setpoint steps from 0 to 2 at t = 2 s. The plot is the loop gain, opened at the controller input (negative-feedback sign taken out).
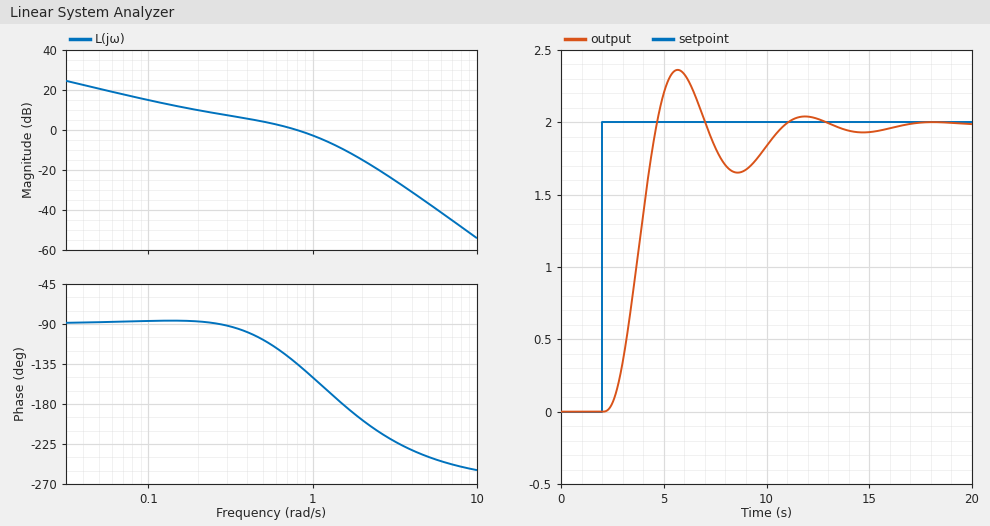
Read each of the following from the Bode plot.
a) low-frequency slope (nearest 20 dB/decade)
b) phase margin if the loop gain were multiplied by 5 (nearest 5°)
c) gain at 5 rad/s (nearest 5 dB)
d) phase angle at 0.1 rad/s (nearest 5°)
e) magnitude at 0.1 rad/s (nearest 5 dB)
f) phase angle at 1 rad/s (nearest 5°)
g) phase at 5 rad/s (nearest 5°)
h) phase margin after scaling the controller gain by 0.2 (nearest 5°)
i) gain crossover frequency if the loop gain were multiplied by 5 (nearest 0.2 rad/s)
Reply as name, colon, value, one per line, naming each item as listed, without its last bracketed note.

low-frequency slope: -20 dB/decade
phase margin if the loop gain were multiplied by 5: -15°
gain at 5 rad/s: -35 dB
phase angle at 0.1 rad/s: -85°
magnitude at 0.1 rad/s: 15 dB
phase angle at 1 rad/s: -150°
phase at 5 rad/s: -240°
phase margin after scaling the controller gain by 0.2: 95°
gain crossover frequency if the loop gain were multiplied by 5: 2.0 rad/s
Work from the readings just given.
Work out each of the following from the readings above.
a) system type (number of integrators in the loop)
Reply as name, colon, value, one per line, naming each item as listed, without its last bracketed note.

system type: 1
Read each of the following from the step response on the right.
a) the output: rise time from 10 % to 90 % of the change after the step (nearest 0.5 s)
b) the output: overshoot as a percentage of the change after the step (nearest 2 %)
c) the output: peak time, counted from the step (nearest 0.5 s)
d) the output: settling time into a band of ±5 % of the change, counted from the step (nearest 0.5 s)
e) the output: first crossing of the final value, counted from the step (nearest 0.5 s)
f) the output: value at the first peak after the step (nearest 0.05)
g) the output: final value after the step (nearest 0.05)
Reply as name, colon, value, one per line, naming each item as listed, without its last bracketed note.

the output: rise time from 10 % to 90 % of the change after the step: 1.5 s
the output: overshoot as a percentage of the change after the step: 18 %
the output: peak time, counted from the step: 3.5 s
the output: settling time into a band of ±5 % of the change, counted from the step: 8.5 s
the output: first crossing of the final value, counted from the step: 2.5 s
the output: value at the first peak after the step: 2.35
the output: final value after the step: 2.00
